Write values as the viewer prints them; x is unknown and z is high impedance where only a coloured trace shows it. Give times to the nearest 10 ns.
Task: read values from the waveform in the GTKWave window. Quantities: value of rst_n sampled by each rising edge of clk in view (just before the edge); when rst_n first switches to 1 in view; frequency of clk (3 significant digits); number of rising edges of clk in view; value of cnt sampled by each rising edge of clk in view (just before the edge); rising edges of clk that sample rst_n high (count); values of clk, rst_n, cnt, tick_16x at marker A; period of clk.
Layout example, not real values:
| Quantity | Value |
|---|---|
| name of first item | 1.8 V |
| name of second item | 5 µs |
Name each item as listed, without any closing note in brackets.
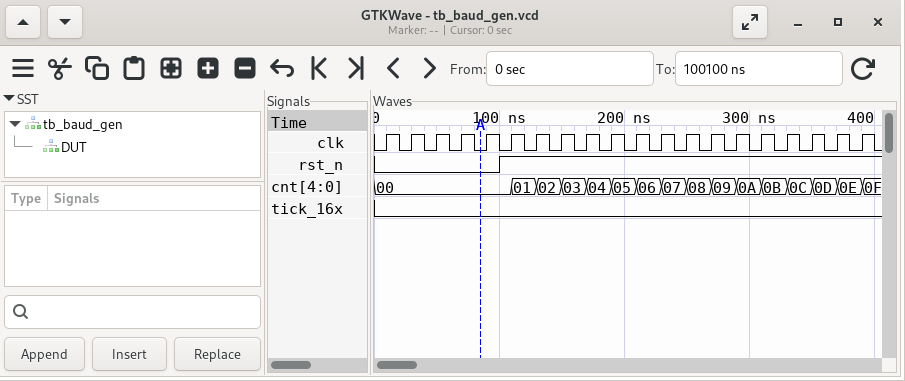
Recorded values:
| Quantity | Value |
|---|---|
| value of rst_n sampled by each rising edge of clk in view | 0 0 0 0 0 1 1 1 1 1 1 1 1 1 1 1 1 1 1 1 |
| when rst_n first switches to 1 in view | 100 ns |
| frequency of clk | 50.0 MHz |
| number of rising edges of clk in view | 20 |
| value of cnt sampled by each rising edge of clk in view | 00, 00, 00, 00, 00, 00, 01, 02, 03, 04, 05, 06, 07, 08, 09, 0A, 0B, 0C, 0D, 0E |
| rising edges of clk that sample rst_n high | 15 |
| values of clk, rst_n, cnt, tick_16x at marker A | clk=0, rst_n=0, cnt=00, tick_16x=0 |
| period of clk | 20 ns |
